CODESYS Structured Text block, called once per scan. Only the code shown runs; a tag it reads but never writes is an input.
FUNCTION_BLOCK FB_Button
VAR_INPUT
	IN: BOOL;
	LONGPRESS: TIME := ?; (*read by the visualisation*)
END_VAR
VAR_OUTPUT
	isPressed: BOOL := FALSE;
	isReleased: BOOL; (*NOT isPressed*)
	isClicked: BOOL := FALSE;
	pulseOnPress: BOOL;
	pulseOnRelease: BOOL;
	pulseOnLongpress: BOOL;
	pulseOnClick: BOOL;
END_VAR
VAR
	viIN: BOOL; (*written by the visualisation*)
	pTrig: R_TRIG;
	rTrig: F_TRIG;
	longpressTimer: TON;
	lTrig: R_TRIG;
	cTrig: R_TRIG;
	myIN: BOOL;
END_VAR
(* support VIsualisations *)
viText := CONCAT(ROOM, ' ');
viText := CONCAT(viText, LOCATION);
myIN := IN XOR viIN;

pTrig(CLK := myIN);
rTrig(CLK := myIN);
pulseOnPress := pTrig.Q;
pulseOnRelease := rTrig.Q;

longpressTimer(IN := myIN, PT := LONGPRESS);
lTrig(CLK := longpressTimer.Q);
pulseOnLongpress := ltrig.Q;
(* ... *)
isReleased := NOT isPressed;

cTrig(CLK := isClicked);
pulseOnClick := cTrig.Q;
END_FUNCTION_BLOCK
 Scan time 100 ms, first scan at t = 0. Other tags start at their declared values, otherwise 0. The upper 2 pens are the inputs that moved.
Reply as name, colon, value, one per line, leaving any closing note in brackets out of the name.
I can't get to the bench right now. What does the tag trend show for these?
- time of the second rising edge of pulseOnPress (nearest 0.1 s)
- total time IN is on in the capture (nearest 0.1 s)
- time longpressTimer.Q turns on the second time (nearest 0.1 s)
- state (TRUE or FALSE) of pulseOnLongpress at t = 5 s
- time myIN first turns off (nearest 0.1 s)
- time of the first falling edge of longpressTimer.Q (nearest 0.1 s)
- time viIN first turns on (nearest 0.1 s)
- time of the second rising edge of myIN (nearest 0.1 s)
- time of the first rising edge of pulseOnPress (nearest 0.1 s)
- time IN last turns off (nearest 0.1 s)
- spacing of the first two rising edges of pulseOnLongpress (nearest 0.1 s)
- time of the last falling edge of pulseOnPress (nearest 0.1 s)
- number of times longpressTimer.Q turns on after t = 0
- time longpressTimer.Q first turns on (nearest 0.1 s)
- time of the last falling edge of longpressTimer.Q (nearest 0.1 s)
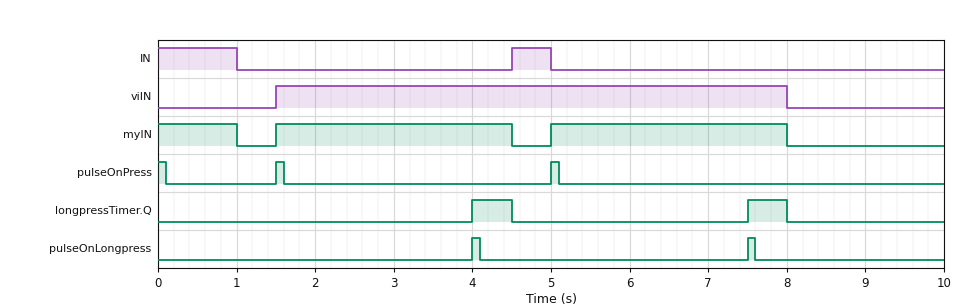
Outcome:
time of the second rising edge of pulseOnPress: 5.0 s
total time IN is on in the capture: 1.5 s
time longpressTimer.Q turns on the second time: 7.5 s
state (TRUE or FALSE) of pulseOnLongpress at t = 5 s: FALSE
time myIN first turns off: 1.0 s
time of the first falling edge of longpressTimer.Q: 4.5 s
time viIN first turns on: 1.5 s
time of the second rising edge of myIN: 5.0 s
time of the first rising edge of pulseOnPress: 1.5 s
time IN last turns off: 5.0 s
spacing of the first two rising edges of pulseOnLongpress: 3.5 s
time of the last falling edge of pulseOnPress: 5.1 s
number of times longpressTimer.Q turns on after t = 0: 2
time longpressTimer.Q first turns on: 4.0 s
time of the last falling edge of longpressTimer.Q: 8.0 s
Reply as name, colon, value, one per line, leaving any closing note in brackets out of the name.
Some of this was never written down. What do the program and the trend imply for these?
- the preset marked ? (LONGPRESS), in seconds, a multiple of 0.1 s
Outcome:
the preset marked ? (LONGPRESS), in seconds, a multiple of 0.1 s: 2.5 s
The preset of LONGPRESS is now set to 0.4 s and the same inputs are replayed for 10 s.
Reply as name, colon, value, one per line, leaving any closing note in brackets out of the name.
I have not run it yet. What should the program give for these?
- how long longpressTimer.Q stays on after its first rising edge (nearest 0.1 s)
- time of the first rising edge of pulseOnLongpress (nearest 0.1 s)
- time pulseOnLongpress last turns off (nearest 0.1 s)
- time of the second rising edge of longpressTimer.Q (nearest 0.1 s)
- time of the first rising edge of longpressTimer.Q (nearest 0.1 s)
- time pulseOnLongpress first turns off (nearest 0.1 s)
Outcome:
how long longpressTimer.Q stays on after its first rising edge: 0.6 s
time of the first rising edge of pulseOnLongpress: 0.4 s
time pulseOnLongpress last turns off: 5.5 s
time of the second rising edge of longpressTimer.Q: 1.9 s
time of the first rising edge of longpressTimer.Q: 0.4 s
time pulseOnLongpress first turns off: 0.5 s
